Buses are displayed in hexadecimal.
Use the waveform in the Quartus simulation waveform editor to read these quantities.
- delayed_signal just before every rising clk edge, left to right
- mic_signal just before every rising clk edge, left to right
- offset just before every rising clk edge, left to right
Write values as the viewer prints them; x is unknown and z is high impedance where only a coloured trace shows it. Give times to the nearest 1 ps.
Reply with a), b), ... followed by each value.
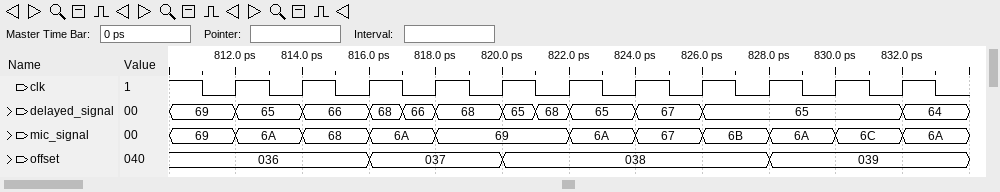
a) 69, 65, 66, 66, 68, 68, 65, 67, 65, 65, 65
b) 69, 6A, 68, 6A, 69, 69, 6A, 67, 6B, 6A, 6C
c) 036, 036, 036, 037, 037, 038, 038, 038, 038, 039, 039
